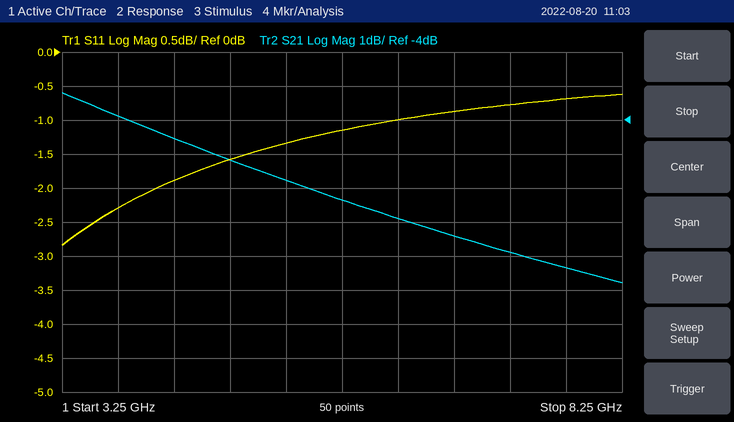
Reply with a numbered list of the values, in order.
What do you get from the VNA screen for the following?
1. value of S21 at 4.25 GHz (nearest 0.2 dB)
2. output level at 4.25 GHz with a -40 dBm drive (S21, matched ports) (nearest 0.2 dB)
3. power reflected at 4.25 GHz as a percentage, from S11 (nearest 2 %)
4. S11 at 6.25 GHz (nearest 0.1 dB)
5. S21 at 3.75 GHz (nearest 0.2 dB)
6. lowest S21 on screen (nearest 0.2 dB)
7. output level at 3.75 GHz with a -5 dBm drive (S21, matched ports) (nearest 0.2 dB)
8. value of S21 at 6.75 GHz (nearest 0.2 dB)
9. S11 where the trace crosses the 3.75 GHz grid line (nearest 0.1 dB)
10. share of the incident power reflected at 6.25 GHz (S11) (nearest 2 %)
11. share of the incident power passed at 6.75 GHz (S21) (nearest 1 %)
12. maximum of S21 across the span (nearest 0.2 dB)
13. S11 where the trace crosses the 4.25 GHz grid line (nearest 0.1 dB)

1. -4.6 dB
2. -44.6 dBm
3. 64 %
4. -1.0 dB
5. -3.8 dB
6. -8.8 dB
7. -8.8 dBm
8. -7.4 dB
9. -2.3 dB
10. 80 %
11. 18 %
12. -3.2 dB
13. -1.9 dB
